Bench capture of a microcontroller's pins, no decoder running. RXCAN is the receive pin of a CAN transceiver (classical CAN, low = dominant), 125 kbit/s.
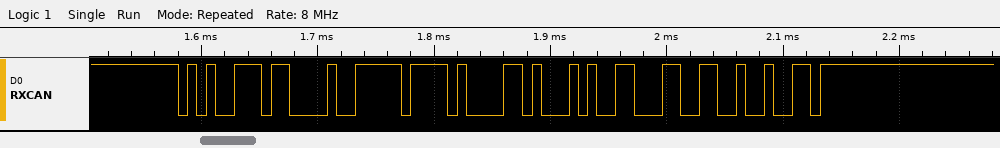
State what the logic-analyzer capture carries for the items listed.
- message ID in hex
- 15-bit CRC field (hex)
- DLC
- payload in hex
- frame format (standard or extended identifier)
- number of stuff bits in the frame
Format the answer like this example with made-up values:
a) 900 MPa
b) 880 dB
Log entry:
a) 0x53B
b) 0x6649
c) 4
d) FF A1 A2 98
e) standard
f) 1
